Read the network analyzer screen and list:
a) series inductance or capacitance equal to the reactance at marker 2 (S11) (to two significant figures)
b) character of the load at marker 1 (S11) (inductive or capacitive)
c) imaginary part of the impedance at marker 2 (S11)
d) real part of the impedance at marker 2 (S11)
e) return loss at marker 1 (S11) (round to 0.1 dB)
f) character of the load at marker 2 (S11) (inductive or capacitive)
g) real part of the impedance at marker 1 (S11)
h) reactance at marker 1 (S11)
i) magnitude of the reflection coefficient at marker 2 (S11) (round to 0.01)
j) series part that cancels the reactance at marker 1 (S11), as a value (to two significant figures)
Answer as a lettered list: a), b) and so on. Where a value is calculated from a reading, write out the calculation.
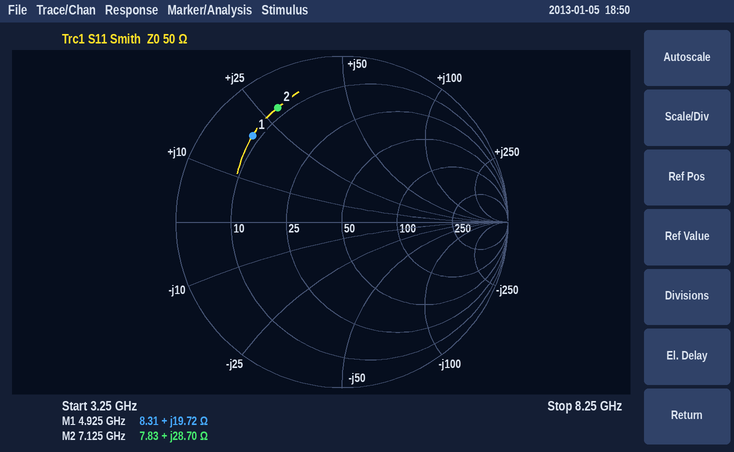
a) L = 28.7 Ω/(2π × 7.125 GHz) ≈ 641 pH, so 640 pH to two significant figures
b) inductive
c) +28.70 Ω
d) 7.83 Ω
e) 2.5 dB
f) inductive
g) 8.31 Ω
h) +19.72 Ω
i) 0.79
j) C = 1/(2π × 4.925 GHz × 19.72 Ω) ≈ 1.6 pF
